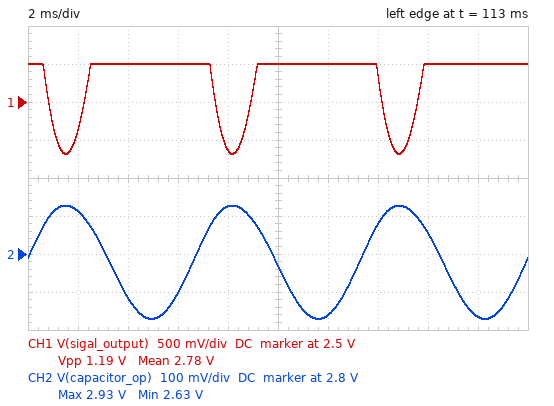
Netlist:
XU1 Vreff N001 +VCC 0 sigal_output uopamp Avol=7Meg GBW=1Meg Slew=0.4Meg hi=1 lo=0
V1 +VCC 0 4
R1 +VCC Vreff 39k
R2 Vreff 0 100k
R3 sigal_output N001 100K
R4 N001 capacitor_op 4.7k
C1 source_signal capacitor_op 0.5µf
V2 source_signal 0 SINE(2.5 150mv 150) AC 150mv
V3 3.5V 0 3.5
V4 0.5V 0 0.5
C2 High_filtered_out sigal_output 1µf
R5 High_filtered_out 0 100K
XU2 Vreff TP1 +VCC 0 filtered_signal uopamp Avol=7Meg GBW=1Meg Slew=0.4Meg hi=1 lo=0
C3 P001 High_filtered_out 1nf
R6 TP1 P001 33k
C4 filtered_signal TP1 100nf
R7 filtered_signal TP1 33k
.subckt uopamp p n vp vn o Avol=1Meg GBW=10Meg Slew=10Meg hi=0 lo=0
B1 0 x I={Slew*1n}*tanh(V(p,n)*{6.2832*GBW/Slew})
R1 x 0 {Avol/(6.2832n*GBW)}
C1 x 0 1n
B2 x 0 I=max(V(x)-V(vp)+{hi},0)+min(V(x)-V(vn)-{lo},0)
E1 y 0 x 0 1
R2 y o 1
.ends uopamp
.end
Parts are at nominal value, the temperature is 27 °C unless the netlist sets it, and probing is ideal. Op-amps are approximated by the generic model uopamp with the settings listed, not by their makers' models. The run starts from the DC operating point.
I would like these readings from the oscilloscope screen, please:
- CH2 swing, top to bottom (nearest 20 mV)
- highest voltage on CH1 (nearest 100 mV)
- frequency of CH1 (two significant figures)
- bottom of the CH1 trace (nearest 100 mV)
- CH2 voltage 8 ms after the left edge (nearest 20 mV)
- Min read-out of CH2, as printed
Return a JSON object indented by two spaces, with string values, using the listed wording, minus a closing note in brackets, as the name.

{
  "CH2 swing, top to bottom": "300 mV",
  "highest voltage on CH1": "3.0 V",
  "frequency of CH1": "150 Hz",
  "bottom of the CH1 trace": "1.8 V",
  "CH2 voltage 8 ms after the left edge": "2.92 V",
  "Min read-out of CH2, as printed": "2.63 V"
}
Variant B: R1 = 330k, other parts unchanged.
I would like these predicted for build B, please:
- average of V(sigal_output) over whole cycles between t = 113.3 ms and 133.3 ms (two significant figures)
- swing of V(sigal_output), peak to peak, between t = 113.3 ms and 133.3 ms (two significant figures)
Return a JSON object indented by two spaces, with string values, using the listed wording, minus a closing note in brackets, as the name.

{
  "average of V(sigal_output) over whole cycles between t = 113.3 ms and 133.3 ms": "970 mV",
  "swing of V(sigal_output), peak to peak, between t = 113.3 ms and 133.3 ms": "3.0 V"
}
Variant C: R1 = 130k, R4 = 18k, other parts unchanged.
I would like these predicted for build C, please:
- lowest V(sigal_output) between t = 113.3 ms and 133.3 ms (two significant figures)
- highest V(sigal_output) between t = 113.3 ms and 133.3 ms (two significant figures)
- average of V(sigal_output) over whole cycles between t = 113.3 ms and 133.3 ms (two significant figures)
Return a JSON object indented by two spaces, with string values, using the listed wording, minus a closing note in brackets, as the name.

{
  "lowest V(sigal_output) between t = 113.3 ms and 133.3 ms": "910 mV",
  "highest V(sigal_output) between t = 113.3 ms and 133.3 ms": "2.6 V",
  "average of V(sigal_output) over whole cycles between t = 113.3 ms and 133.3 ms": "1.7 V"
}
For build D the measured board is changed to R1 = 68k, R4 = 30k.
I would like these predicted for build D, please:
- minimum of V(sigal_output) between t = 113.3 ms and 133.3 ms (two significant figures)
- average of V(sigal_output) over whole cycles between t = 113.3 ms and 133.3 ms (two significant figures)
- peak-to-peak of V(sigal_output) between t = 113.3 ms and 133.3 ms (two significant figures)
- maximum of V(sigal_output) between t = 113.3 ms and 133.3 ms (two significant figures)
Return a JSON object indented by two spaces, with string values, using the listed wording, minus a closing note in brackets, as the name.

{
  "minimum of V(sigal_output) between t = 113.3 ms and 133.3 ms": "1.9 V",
  "average of V(sigal_output) over whole cycles between t = 113.3 ms and 133.3 ms": "2.4 V",
  "peak-to-peak of V(sigal_output) between t = 113.3 ms and 133.3 ms": "1.0 V",
  "maximum of V(sigal_output) between t = 113.3 ms and 133.3 ms": "2.9 V"
}
